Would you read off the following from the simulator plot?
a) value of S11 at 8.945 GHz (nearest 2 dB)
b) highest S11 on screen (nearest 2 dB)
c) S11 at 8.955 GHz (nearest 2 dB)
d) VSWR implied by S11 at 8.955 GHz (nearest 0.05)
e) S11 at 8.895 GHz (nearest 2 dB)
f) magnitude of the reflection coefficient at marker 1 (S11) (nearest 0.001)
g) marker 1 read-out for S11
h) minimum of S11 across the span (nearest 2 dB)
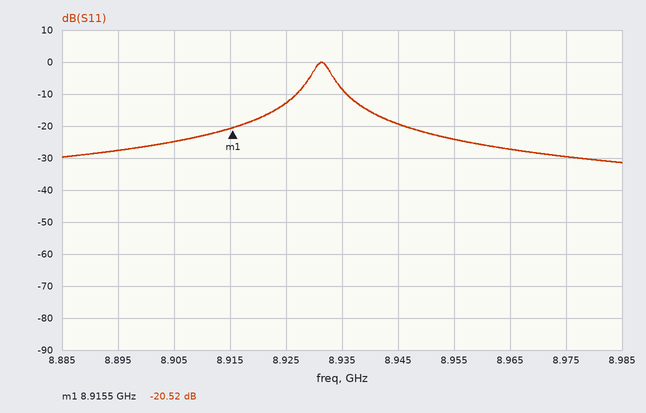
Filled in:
-20 dB
0 dB
-24 dB
1.15
-28 dB
0.094
-20.52 dB
-32 dB
